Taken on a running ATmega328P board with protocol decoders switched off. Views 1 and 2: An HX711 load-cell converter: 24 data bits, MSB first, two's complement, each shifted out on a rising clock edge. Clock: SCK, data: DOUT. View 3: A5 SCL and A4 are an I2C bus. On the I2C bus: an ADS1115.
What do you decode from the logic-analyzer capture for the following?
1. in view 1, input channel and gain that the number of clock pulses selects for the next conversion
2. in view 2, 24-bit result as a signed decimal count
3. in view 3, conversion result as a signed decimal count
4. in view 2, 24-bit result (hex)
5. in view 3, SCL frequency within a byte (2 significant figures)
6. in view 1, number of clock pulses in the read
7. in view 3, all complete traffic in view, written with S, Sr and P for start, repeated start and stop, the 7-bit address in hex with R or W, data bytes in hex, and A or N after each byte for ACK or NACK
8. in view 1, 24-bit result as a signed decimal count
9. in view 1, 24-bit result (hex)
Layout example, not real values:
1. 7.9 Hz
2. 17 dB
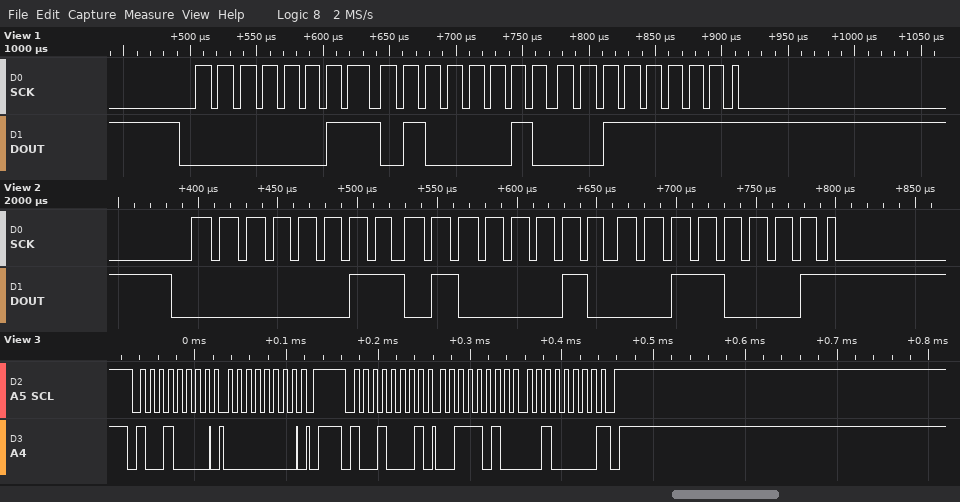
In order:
1. channel A, gain 128
2. 213553
3. 14880
4. 0x034231
5. 100 kHz
6. 25
7. S 48W A 00 A P S 48R A 3A A 20 N P
8. 213567
9. 0x03423F
